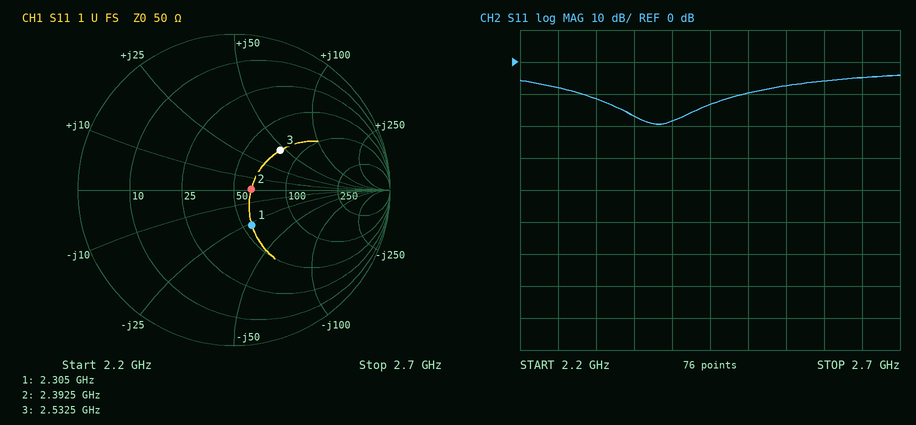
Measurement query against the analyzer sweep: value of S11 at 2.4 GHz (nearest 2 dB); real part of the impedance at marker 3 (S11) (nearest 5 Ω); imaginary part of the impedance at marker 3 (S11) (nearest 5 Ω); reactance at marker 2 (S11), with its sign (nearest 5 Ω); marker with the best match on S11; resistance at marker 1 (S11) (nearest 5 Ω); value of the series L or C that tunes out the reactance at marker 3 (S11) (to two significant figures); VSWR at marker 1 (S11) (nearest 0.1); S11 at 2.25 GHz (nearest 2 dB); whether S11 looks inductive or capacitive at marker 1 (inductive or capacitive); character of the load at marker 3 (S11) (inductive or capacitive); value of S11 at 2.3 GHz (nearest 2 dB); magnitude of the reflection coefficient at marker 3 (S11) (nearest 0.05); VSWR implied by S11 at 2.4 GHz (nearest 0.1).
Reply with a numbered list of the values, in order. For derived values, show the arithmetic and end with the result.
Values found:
1. -18 dB
2. 75 Ω
3. +45 Ω
4. 0 Ω
5. marker 2
6. 55 Ω
7. C = 1/(2π × 2.5325 GHz × 45 Ω) ≈ 1.4 pF
8. 1.7
9. -8 dB
10. capacitive
11. inductive
12. -12 dB
13. 0.40
14. |Γ| = 10^(-18/20) = 0.1259; VSWR = (1 + 0.1259)/(1 − 0.1259) ≈ 1.3
